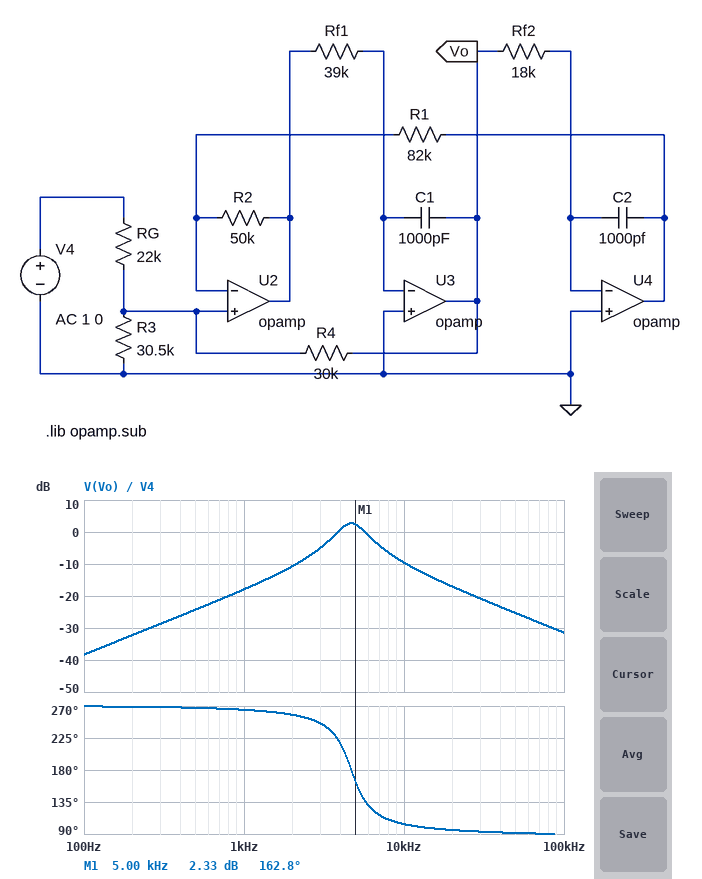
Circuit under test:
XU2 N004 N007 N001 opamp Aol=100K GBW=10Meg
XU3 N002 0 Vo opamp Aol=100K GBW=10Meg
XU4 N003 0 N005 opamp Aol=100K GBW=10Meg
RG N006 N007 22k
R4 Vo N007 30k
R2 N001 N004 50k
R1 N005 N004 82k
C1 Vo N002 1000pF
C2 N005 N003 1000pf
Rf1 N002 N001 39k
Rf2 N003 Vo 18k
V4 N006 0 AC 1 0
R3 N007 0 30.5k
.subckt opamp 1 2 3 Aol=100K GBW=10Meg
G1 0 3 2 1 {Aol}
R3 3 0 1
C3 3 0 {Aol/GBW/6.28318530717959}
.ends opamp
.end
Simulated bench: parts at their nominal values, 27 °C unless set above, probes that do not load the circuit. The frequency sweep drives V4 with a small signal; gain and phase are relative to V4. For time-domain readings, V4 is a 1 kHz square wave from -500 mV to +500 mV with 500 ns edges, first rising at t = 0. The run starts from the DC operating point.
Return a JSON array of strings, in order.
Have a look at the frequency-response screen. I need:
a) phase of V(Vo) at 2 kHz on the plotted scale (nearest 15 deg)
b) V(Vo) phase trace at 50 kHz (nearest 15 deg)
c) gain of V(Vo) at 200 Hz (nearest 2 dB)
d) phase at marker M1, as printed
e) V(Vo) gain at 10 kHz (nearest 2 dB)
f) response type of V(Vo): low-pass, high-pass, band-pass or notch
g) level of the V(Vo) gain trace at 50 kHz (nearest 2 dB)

["255 deg", "90 deg", "-32 dB", "162.8 deg", "-10 dB", "band-pass", "-26 dB"]
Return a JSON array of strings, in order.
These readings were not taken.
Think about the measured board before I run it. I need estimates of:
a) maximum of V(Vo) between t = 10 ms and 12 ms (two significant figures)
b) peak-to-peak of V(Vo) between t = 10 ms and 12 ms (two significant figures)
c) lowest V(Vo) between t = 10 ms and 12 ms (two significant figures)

["430 mV", "860 mV", "-430 mV"]
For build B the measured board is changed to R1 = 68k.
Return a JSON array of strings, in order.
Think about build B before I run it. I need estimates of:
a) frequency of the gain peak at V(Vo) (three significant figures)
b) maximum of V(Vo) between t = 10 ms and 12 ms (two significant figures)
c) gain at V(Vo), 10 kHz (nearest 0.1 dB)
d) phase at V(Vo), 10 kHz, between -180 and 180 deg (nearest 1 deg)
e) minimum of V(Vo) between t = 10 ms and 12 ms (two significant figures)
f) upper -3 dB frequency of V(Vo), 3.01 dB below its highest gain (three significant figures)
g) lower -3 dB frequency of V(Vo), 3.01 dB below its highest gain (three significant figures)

["5.15 kHz", "440 mV", "-8.5 dB", "106 deg", "-440 mV", "6.31 kHz", "4.20 kHz"]
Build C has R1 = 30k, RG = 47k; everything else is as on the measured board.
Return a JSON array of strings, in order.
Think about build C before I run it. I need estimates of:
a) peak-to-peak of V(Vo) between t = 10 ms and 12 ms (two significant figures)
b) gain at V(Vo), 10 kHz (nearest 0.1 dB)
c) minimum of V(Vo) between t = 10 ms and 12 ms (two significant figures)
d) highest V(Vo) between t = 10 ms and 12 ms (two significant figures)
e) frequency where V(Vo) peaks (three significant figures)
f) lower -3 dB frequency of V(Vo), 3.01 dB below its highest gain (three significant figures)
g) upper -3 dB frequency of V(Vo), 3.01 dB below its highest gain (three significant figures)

["480 mV", "-6.7 dB", "-240 mV", "240 mV", "7.76 kHz", "5.96 kHz", "10.1 kHz"]
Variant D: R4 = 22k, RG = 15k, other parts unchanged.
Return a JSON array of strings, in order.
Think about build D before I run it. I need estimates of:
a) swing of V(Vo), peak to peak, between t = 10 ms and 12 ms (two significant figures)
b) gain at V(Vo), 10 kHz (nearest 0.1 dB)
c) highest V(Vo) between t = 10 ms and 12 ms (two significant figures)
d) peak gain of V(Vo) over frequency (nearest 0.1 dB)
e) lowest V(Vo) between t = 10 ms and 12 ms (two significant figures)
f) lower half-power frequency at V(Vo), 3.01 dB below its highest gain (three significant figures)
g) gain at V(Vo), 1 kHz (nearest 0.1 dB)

["950 mV", "-8.5 dB", "480 mV", "3.4 dB", "-480 mV", "3.77 kHz", "-16.9 dB"]
